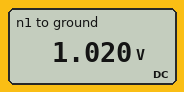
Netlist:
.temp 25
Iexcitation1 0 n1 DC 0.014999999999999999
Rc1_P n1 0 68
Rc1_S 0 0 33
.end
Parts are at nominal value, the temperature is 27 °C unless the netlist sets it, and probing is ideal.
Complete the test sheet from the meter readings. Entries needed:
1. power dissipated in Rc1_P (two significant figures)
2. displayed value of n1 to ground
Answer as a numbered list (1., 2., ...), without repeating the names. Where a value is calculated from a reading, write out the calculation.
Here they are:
1. (1.02 V)^2 / 68 Ω = 15 mW
2. 1.020 V
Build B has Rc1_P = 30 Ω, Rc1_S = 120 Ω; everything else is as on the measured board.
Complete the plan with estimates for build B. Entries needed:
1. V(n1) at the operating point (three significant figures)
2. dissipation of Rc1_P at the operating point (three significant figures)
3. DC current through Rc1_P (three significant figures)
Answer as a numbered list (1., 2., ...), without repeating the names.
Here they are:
1. 450 mV
2. 6.75 mW
3. 15.0 mA
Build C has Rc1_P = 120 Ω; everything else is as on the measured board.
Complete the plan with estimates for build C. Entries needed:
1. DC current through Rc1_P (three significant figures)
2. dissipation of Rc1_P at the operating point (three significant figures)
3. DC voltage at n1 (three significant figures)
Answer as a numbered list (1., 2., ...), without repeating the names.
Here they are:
1. 15.0 mA
2. 27.0 mW
3. 1.80 V
